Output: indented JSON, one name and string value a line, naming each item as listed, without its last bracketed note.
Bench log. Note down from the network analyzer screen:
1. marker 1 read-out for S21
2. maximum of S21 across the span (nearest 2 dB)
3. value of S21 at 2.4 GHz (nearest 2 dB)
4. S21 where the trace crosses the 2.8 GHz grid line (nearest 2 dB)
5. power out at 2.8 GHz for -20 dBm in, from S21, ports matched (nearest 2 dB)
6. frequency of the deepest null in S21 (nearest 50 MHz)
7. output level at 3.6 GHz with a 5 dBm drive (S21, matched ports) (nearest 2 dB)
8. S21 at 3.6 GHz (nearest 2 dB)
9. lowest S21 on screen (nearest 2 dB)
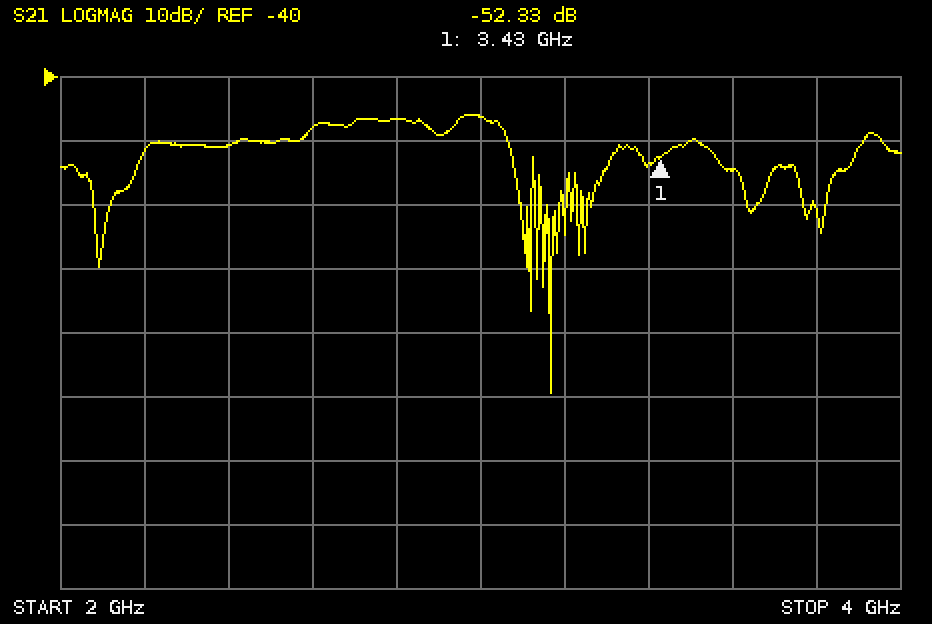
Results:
{
  "marker 1 read-out for S21": "-52.33 dB",
  "maximum of S21 across the span": "-46 dB",
  "value of S21 at 2.4 GHz": "-50 dB",
  "S21 where the trace crosses the 2.8 GHz grid line": "-46 dB",
  "power out at 2.8 GHz for -20 dBm in, from S21, ports matched": "-66 dBm",
  "frequency of the deepest null in S21": "3.15 GHz",
  "output level at 3.6 GHz with a 5 dBm drive (S21, matched ports)": "-50 dBm",
  "S21 at 3.6 GHz": "-54 dB",
  "lowest S21 on screen": "-90 dB"
}
